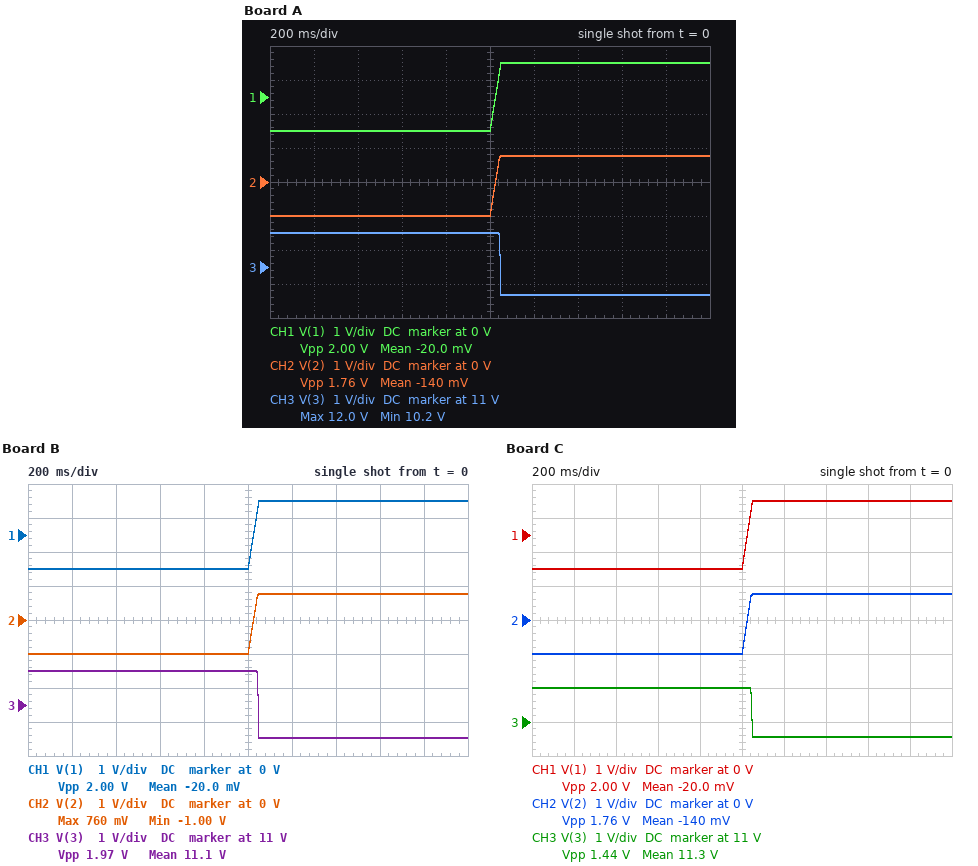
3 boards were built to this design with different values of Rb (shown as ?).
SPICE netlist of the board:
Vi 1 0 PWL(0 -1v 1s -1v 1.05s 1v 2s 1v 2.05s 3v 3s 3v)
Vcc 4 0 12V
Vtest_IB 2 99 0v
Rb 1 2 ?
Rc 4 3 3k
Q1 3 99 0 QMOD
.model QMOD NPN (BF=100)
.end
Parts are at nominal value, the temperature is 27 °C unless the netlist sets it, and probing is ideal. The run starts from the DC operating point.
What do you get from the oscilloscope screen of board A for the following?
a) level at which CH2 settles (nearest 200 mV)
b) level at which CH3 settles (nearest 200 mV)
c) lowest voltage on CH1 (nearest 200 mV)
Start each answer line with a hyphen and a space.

- 800 mV
- 10.2 V
- -1.0 V
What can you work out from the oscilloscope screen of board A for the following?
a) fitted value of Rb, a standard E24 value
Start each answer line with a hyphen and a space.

- 39 kΩ
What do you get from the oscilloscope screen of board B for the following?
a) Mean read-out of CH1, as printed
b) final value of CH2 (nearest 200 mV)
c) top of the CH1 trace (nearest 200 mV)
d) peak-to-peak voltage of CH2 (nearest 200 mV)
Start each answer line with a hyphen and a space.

- -20.0 mV
- 800 mV
- 1.0 V
- 1.8 V
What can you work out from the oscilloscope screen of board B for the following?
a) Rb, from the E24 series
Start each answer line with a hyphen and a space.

- 36 kΩ
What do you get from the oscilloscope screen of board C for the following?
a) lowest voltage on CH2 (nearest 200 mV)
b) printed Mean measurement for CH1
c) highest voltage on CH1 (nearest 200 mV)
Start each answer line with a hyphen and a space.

- -1.0 V
- -20.0 mV
- 1.0 V
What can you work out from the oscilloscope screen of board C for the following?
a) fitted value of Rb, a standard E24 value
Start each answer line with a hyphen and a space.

- 51 kΩ
